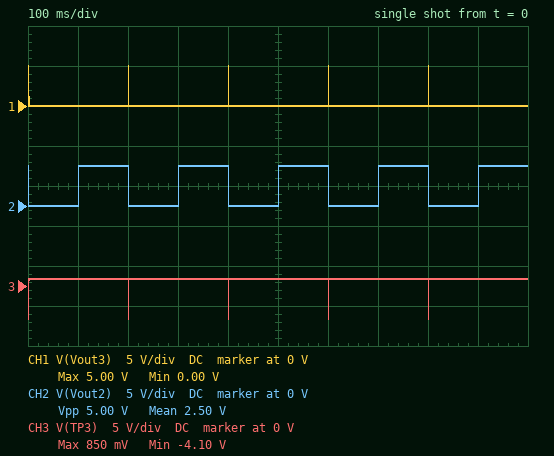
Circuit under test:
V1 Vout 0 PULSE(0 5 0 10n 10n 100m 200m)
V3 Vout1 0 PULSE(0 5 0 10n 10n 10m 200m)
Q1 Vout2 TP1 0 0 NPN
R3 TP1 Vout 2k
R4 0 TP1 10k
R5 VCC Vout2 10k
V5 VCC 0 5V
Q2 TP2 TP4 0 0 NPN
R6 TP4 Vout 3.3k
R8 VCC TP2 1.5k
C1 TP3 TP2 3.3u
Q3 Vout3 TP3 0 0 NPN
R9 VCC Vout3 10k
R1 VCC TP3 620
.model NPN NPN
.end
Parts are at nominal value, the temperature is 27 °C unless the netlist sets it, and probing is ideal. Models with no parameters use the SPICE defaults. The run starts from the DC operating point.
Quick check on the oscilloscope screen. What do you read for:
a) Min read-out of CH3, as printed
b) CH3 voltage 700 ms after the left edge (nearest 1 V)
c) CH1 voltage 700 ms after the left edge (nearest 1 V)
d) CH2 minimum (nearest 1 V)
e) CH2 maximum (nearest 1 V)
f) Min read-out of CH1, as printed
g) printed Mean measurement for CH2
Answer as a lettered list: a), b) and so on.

a) -4.10 V
b) 1 V
c) 0 V
d) 0 V
e) 5 V
f) 0.00 V
g) 2.50 V
